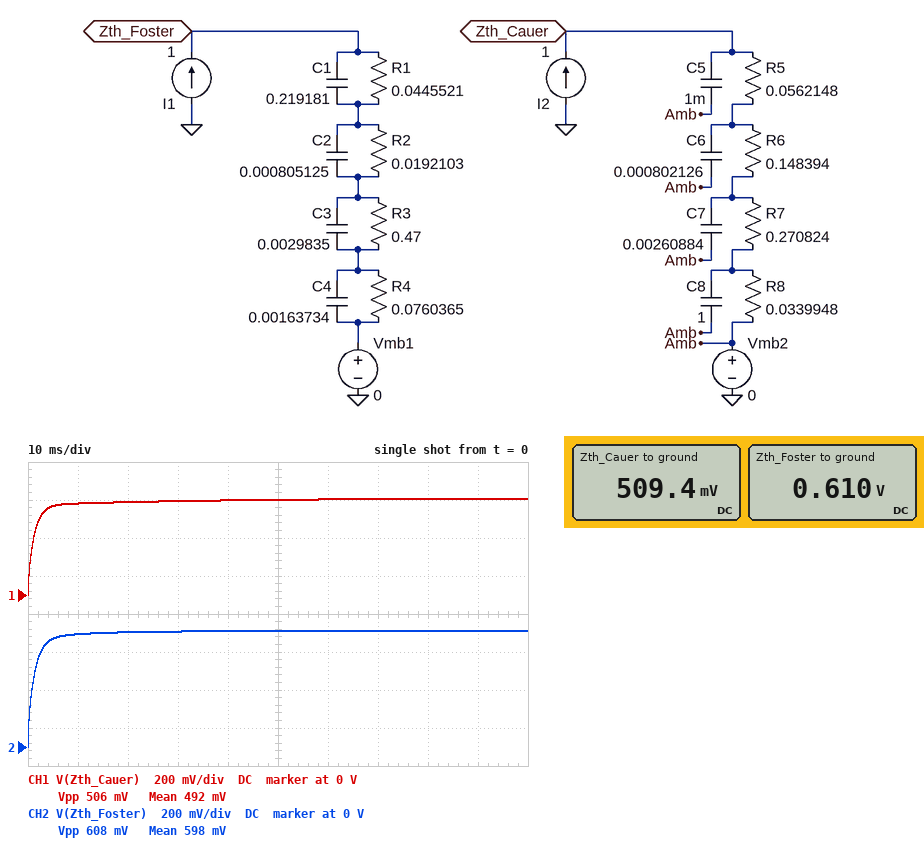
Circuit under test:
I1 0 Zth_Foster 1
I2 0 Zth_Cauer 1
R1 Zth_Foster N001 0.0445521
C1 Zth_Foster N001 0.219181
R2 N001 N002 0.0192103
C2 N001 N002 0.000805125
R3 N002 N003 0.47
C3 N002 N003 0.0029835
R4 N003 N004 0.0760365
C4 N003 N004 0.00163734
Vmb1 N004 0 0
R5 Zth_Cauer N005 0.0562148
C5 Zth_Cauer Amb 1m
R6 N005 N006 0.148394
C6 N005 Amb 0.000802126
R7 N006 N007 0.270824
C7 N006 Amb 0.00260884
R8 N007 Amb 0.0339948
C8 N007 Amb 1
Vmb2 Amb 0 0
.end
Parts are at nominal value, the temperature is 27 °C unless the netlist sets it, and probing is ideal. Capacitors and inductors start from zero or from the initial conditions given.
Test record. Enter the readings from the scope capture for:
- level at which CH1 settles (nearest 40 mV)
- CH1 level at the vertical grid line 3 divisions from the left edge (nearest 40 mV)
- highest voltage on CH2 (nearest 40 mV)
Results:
520 mV
480 mV
600 mV
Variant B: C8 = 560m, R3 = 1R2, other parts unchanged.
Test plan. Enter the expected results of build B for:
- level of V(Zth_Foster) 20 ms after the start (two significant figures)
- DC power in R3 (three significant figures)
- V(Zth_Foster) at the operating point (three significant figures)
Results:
1.3 V
1.20 W
1.34 V
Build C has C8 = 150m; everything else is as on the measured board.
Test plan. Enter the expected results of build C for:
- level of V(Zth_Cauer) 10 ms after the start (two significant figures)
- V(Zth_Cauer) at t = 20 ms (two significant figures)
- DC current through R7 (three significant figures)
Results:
500 mV
510 mV
1.00 A
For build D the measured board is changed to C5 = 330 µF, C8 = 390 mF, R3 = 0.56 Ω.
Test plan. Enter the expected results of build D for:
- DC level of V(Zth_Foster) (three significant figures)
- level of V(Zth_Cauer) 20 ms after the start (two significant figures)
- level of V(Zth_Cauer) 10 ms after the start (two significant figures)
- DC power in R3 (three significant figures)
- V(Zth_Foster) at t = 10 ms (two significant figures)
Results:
700 mV
500 mV
490 mV
560 mW
680 mV
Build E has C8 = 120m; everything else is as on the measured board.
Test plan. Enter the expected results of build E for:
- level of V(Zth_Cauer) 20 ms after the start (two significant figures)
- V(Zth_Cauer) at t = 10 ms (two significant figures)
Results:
510 mV
500 mV
